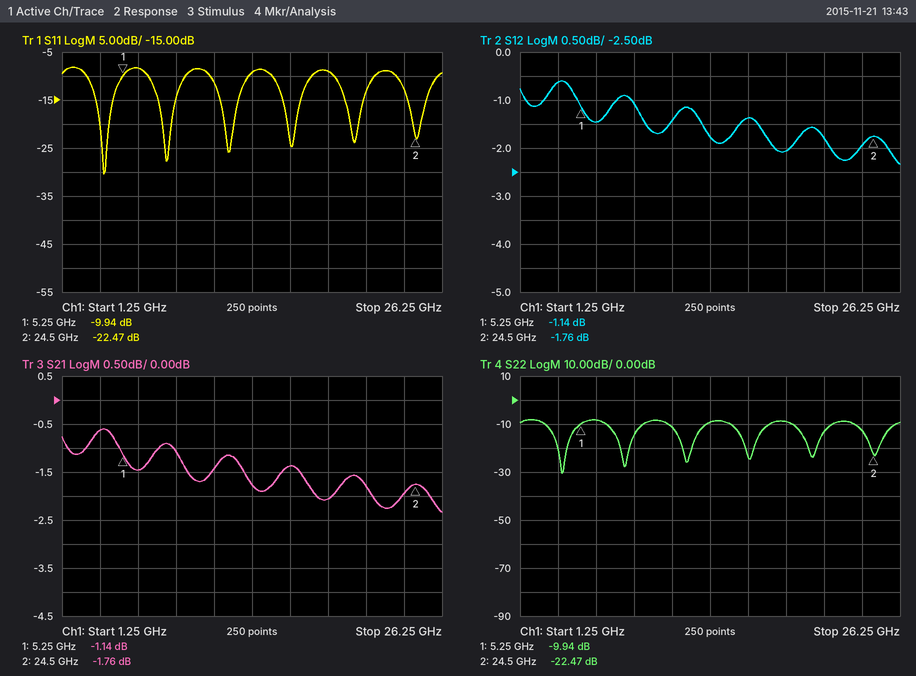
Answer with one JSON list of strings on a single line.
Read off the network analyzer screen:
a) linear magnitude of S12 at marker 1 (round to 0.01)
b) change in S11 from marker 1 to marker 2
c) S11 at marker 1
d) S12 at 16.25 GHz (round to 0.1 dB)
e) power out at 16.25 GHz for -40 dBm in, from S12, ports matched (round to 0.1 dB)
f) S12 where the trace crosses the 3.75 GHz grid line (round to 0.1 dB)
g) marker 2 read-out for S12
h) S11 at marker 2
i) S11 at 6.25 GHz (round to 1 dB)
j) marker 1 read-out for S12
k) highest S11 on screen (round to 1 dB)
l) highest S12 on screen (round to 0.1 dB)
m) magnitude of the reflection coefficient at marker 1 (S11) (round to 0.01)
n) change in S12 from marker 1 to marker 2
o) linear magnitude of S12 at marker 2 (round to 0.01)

["0.88", "-12.53 dB", "-9.94 dB", "-1.4 dB", "-41.4 dBm", "-0.6 dB", "-1.76 dB", "-22.47 dB", "-8 dB", "-1.14 dB", "-8 dB", "-0.6 dB", "0.32", "-0.62 dB", "0.82"]
